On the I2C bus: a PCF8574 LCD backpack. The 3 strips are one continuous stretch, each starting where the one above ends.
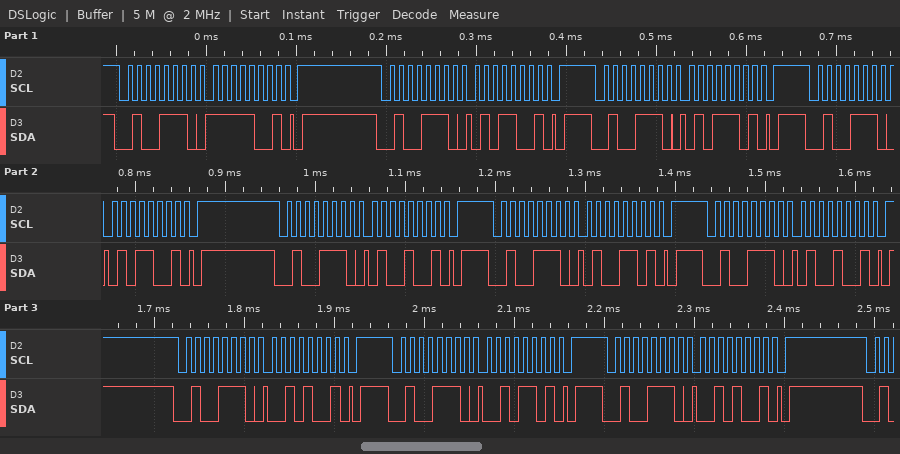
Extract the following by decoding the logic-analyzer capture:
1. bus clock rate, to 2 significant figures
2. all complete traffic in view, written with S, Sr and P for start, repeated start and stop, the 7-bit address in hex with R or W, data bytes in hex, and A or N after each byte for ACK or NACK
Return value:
100 kHz
S 27W A F9 A P S 27W A 59 A P S 27W A 5D A P S 27W A 59 A P S 27W A 49 A P S 27W A 4D A P S 27W A 49 A P S 27W A 29 A P S 27W A 2D A P S 27W A 29 A P
